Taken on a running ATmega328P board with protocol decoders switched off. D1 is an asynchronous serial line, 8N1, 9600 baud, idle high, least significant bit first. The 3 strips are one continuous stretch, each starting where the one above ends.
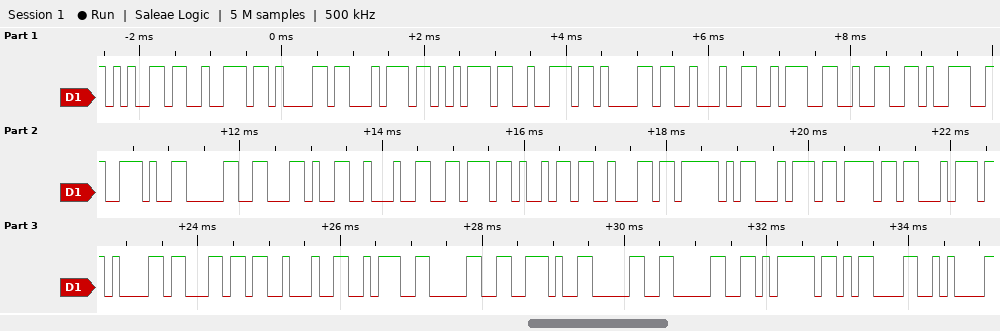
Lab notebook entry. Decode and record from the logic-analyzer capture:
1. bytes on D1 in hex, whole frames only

65 72 61 74 75 72 61 22 3A 32 39 2E 30 2C 22 76 69 62 5F 74 6F 74 61 6C 22 3A 30 2E 30 30 7D 0D 0A
